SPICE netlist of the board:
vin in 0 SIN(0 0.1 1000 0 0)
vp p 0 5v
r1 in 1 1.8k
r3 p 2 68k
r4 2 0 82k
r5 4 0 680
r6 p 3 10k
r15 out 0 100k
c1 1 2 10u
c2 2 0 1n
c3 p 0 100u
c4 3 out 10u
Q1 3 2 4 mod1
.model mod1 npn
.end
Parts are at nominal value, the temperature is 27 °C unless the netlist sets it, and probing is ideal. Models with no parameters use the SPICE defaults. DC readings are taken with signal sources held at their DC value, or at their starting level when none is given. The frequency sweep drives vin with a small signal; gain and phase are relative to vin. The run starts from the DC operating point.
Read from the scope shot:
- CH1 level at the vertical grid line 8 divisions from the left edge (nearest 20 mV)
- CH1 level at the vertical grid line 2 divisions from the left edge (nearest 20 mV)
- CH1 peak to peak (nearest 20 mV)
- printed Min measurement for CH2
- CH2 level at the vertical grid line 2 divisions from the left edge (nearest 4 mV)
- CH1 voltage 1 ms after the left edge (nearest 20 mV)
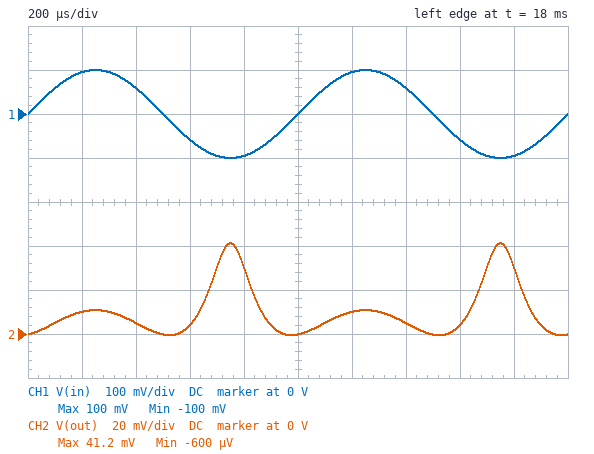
-60 mV
60 mV
200 mV
-600 µV
4 mV
0 V
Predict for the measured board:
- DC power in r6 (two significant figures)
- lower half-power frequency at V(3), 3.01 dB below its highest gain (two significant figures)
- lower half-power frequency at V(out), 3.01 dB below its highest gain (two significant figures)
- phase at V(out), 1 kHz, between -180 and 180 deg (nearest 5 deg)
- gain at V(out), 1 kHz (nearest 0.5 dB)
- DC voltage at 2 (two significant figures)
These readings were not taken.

2.1 mW
6.2 Hz
6.2 Hz
0 deg
-27.5 dB
1.1 V
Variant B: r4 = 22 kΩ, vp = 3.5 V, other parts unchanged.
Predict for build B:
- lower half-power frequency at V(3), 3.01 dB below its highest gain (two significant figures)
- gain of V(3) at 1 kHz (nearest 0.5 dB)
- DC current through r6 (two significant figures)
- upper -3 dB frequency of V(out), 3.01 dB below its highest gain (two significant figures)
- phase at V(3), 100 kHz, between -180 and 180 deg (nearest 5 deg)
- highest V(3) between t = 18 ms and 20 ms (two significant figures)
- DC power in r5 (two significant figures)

1.0 Hz
19.5 dB
150 µA
100 kHz
135 deg
2.8 V
16 µW
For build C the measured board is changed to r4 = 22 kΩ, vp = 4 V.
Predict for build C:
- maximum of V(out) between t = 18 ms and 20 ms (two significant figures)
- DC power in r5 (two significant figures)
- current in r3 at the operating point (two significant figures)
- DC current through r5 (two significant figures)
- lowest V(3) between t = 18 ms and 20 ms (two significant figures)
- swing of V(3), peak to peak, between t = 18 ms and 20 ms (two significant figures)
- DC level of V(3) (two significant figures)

1.0 V
53 µW
45 µA
280 µA
370 mV
1.9 V
1.2 V
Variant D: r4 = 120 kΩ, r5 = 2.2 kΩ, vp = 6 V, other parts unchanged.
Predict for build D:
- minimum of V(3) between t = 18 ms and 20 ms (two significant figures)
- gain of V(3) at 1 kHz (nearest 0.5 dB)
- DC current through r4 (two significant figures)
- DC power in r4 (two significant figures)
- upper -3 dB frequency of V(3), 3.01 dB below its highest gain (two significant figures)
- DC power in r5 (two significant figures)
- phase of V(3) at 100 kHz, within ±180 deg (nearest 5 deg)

1.2 V
-9.5 dB
16 µA
30 µW
170 kHz
600 µW
-30 deg
